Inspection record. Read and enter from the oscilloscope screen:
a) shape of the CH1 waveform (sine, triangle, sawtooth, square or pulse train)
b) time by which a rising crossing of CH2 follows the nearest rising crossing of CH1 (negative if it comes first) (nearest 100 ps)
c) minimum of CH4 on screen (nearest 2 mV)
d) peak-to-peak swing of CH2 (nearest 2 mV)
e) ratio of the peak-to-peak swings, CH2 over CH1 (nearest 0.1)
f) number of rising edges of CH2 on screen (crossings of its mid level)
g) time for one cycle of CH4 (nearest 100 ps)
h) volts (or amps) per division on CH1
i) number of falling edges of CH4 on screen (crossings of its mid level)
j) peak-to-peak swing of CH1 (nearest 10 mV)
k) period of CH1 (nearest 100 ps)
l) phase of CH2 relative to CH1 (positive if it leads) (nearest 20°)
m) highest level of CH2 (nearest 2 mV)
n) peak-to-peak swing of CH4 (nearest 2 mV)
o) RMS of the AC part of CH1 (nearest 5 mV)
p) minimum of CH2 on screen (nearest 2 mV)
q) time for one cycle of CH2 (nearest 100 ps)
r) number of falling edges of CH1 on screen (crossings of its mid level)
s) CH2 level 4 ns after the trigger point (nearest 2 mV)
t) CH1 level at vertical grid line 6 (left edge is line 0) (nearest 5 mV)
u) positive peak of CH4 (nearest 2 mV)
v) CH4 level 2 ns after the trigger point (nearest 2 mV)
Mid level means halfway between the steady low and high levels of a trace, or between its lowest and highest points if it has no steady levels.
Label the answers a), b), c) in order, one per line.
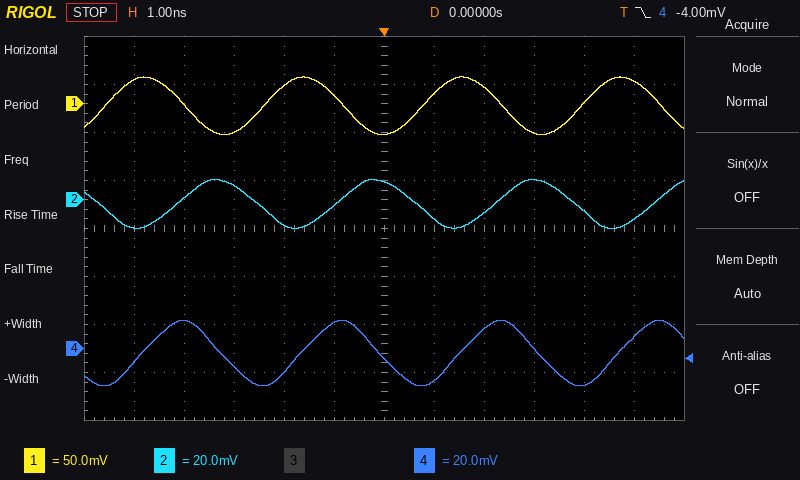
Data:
a) sine
b) +1.4 ns
c) -16 mV
d) 20 mV
e) 0.3
f) 4
g) 3.2 ns
h) 50 mV
i) 3
j) 60 mV
k) 3.2 ns
l) -160°
m) 8 mV
n) 28 mV
o) 20 mV
p) -12 mV
q) 3.2 ns
r) 4
s) -4 mV
t) -30 mV
u) 12 mV
v) 8 mV
